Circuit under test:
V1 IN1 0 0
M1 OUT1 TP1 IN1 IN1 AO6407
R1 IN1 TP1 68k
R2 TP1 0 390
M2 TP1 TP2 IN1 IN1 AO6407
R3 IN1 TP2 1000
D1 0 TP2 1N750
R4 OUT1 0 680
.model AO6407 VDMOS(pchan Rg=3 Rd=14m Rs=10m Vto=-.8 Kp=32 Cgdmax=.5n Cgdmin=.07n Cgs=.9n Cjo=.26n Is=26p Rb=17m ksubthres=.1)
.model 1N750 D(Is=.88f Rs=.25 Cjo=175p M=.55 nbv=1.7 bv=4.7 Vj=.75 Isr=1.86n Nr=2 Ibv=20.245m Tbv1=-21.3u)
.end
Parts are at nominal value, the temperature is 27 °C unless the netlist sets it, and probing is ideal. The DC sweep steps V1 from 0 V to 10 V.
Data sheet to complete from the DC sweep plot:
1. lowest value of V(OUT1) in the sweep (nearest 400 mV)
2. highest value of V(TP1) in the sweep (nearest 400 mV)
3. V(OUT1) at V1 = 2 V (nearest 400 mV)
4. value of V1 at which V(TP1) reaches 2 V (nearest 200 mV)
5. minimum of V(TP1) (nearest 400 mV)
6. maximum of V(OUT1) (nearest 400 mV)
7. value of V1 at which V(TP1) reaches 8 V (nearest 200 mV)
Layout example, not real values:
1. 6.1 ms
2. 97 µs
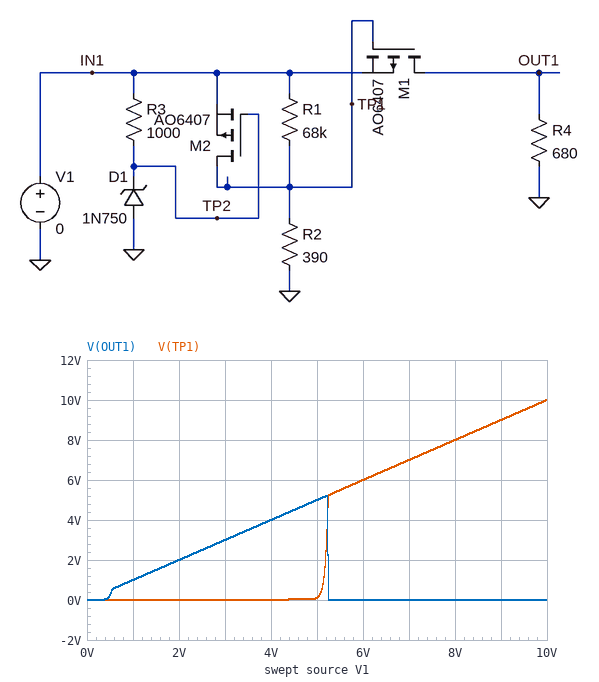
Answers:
1. 0 V
2. 10.0 V
3. 2.0 V
4. 5.2 V
5. 0 V
6. 5.2 V
7. 8.0 V
